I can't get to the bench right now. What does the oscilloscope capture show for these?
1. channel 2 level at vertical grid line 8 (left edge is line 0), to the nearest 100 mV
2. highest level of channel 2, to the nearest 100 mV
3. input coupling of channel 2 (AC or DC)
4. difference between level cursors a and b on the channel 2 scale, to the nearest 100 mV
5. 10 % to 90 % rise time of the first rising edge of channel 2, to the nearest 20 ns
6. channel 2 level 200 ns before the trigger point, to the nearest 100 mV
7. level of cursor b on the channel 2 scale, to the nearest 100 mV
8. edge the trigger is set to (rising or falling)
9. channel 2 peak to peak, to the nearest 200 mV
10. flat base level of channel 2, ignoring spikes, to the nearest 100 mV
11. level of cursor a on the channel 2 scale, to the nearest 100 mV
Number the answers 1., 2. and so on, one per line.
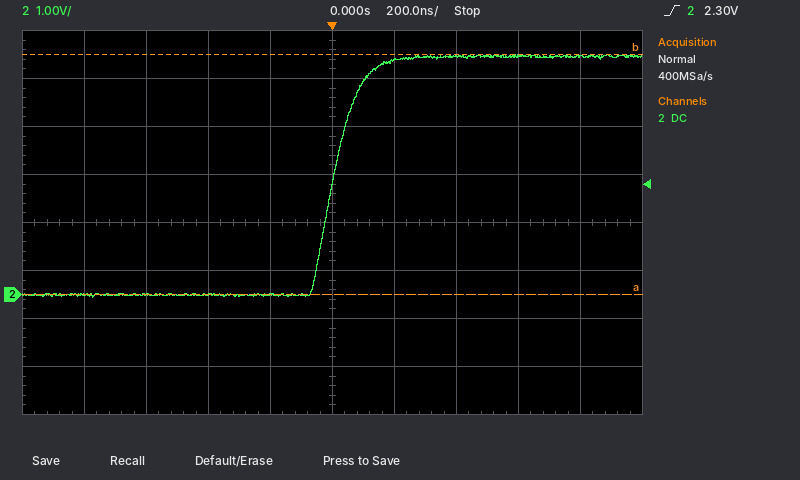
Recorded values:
1. 5.0 V
2. 5.0 V
3. DC
4. 5.0 V
5. 160 ns
6. 0.0 V
7. 5.0 V
8. rising
9. 5.0 V
10. 0.0 V
11. 0.0 V
